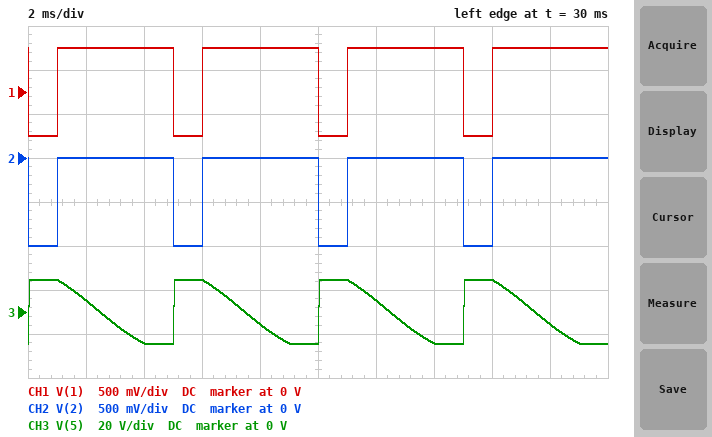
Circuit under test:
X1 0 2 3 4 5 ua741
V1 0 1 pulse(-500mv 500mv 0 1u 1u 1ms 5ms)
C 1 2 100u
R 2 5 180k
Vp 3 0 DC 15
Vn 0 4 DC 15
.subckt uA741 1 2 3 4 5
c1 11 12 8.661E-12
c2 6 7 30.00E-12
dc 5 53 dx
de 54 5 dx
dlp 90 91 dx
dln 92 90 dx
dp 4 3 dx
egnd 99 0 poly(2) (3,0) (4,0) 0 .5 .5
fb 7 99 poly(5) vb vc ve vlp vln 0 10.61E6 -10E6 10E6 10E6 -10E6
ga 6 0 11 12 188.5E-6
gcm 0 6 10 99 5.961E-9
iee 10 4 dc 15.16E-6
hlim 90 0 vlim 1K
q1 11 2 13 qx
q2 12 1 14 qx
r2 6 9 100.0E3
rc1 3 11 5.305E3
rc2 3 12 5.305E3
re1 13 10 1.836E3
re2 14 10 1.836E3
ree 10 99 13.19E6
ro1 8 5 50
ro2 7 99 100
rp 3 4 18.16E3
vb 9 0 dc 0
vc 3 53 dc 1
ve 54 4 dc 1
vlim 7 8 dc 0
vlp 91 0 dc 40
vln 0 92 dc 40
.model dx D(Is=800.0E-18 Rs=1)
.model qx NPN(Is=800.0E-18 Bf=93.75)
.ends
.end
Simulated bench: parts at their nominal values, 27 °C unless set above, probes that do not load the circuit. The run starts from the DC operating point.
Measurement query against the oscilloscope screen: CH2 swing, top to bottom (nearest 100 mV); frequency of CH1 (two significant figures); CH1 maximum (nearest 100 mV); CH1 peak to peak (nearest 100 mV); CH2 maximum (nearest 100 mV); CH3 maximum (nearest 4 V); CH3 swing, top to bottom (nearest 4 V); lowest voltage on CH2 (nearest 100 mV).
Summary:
1.0 V
200 Hz
500 mV
1.0 V
0 V
16 V
28 V
-1.0 V
